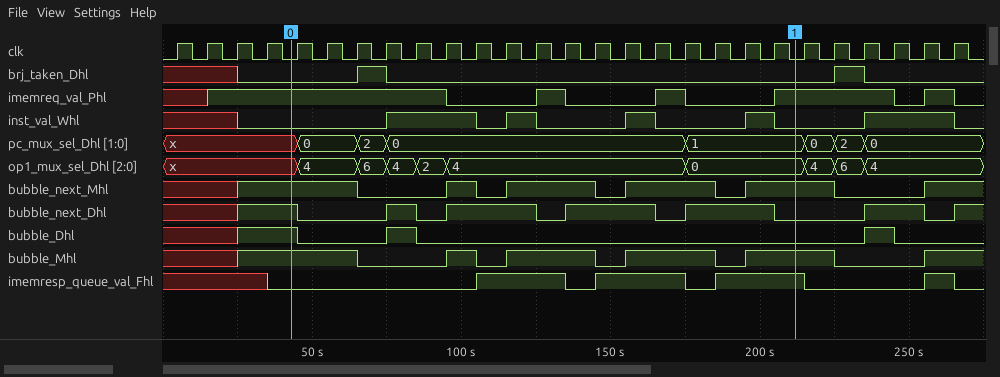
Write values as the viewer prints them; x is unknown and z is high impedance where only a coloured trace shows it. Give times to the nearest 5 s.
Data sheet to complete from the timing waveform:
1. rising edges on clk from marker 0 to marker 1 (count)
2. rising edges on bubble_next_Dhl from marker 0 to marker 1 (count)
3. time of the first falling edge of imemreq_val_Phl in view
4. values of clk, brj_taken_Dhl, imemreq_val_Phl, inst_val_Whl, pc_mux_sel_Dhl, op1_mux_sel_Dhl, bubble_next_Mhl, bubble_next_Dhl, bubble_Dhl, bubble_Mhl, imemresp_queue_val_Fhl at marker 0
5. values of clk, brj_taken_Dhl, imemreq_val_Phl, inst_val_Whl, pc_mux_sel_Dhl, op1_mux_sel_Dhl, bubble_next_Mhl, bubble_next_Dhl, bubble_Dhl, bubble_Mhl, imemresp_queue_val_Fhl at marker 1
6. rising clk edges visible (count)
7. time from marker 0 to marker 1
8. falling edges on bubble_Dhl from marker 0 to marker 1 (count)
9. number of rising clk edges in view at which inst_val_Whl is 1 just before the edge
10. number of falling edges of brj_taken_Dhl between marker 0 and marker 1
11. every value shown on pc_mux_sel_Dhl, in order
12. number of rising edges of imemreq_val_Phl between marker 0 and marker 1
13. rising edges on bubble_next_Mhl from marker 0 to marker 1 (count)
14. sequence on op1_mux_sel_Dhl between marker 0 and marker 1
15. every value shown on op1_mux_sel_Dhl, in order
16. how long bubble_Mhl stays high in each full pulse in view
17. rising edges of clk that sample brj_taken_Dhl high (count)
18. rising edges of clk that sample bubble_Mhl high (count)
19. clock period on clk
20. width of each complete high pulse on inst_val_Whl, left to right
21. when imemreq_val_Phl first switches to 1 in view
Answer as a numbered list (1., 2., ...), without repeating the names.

1. 17
2. 4
3. 95 s
4. clk=0, brj_taken_Dhl=0, imemreq_val_Phl=1, inst_val_Whl=0, pc_mux_sel_Dhl=x, op1_mux_sel_Dhl=x, bubble_next_Mhl=1, bubble_next_Dhl=1, bubble_Dhl=1, bubble_Mhl=1, imemresp_queue_val_Fhl=0
5. clk=0, brj_taken_Dhl=0, imemreq_val_Phl=1, inst_val_Whl=0, pc_mux_sel_Dhl=1, op1_mux_sel_Dhl=0, bubble_next_Mhl=1, bubble_next_Dhl=0, bubble_Dhl=0, bubble_Mhl=1, imemresp_queue_val_Fhl=1
6. 27
7. 170 s
8. 2
9. 9
10. 1
11. x, 0, 2, 0, 1, 0, 2, 0
12. 3
13. 4
14. x, 4, 6, 4, 2, 4, 0
15. x, 4, 6, 4, 2, 4, 0, 4, 6, 4
16. 10 s, 30 s, 30 s, 30 s
17. 2
18. 15
19. 10 s
20. 30 s, 10 s, 10 s, 10 s, 30 s
21. 15 s
